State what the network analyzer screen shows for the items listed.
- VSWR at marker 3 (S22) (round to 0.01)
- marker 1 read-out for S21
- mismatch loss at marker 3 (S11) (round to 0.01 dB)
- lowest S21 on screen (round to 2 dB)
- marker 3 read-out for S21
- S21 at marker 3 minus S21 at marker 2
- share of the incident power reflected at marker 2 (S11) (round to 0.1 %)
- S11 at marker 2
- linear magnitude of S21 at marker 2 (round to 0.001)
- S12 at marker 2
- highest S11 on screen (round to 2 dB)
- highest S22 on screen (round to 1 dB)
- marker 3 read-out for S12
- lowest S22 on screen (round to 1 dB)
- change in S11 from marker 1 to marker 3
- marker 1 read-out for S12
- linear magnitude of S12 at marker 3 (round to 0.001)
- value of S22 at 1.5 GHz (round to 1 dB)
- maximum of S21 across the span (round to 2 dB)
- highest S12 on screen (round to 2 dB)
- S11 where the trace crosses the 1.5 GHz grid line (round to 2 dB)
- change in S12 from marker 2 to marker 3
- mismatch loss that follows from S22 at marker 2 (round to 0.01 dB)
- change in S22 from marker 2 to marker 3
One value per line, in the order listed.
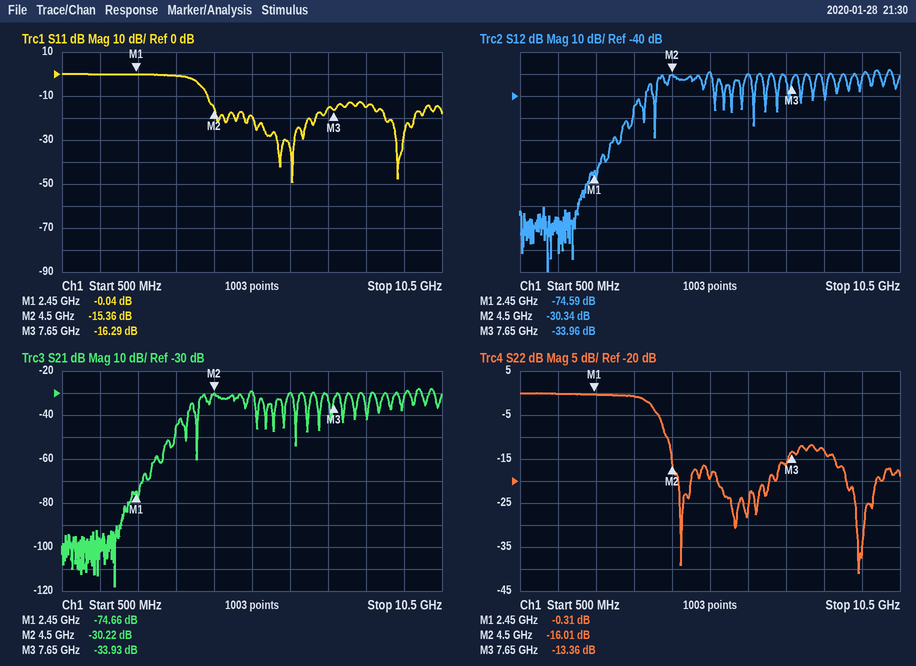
1.55
-74.66 dB
0.10 dB
-118 dB
-33.93 dB
-3.71 dB
2.9 %
-15.36 dB
0.031
-30.34 dB
0 dB
0 dB
-33.96 dB
-41 dB
-16.25 dB
-74.59 dB
0.020
0 dB
-28 dB
-28 dB
0 dB
-3.62 dB
0.11 dB
2.65 dB
